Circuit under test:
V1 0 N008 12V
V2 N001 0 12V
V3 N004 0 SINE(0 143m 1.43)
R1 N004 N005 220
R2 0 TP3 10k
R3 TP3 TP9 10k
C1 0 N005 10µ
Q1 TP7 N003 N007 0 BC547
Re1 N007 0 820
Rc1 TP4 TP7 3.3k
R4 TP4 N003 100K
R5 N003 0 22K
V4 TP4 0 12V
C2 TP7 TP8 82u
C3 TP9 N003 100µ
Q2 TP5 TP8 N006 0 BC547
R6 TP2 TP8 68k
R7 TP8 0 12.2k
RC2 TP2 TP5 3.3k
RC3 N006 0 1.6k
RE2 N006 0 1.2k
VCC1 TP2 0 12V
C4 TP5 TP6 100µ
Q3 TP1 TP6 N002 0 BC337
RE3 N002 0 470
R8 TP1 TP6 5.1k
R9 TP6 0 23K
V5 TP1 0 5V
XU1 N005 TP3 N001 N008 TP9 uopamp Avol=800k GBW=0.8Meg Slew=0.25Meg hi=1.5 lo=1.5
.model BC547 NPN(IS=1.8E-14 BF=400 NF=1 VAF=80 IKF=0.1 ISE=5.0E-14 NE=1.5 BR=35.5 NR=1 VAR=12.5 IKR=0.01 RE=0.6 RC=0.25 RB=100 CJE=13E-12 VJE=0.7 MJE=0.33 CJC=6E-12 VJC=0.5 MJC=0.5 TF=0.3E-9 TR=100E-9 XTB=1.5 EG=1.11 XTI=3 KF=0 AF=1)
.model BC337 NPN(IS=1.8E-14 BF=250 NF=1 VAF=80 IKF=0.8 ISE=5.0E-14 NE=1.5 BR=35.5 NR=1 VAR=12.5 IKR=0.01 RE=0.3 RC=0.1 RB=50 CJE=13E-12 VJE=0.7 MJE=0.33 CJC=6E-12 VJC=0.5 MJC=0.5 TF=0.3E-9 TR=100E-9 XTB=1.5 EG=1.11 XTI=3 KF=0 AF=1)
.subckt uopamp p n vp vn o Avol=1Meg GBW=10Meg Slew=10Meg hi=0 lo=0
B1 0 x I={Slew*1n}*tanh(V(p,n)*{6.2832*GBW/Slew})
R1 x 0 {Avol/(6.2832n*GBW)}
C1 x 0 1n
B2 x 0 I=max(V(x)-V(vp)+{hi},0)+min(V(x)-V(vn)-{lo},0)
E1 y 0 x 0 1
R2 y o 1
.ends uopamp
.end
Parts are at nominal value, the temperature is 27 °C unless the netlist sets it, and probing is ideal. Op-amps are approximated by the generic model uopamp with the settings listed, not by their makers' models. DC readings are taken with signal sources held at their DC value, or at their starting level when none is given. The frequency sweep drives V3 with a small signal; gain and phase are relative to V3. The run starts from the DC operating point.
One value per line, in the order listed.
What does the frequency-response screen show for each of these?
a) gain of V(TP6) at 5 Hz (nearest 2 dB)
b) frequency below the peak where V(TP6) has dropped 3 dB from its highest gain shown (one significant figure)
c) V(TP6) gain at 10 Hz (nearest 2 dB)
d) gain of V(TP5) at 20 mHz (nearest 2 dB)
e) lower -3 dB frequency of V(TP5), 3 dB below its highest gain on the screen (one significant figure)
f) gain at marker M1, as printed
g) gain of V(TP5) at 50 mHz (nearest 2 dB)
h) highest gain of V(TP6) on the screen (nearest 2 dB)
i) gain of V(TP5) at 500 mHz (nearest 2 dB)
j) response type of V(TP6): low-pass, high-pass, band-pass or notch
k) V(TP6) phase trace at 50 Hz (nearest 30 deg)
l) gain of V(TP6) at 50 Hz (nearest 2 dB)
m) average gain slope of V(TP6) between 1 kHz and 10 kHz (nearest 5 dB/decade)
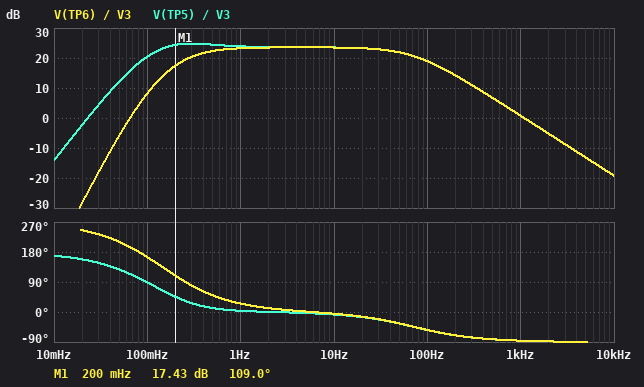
24 dB
300 mHz
24 dB
-2 dB
100 mHz
17.43 dB
12 dB
24 dB
24 dB
band-pass
-30 deg
22 dB
-20 dB/decade
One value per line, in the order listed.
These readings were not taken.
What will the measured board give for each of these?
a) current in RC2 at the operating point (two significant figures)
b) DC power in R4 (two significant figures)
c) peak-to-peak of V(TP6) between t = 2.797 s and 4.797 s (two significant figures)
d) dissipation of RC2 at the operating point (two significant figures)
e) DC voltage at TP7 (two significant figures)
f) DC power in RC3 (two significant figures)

1.6 mA
990 µW
3.9 V
8.7 mW
6.3 V
780 µW
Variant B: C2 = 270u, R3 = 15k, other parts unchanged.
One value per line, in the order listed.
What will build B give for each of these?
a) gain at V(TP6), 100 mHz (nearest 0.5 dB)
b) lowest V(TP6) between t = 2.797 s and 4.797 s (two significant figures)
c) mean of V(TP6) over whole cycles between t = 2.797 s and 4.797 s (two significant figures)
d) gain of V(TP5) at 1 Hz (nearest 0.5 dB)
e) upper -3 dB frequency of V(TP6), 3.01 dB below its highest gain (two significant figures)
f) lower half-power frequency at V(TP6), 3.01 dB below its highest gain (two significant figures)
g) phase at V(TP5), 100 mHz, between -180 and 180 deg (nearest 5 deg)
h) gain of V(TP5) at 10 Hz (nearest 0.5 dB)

14.5 dB
1.2 V
3.7 V
26.0 dB
73 Hz
260 mHz
55 deg
25.5 dB
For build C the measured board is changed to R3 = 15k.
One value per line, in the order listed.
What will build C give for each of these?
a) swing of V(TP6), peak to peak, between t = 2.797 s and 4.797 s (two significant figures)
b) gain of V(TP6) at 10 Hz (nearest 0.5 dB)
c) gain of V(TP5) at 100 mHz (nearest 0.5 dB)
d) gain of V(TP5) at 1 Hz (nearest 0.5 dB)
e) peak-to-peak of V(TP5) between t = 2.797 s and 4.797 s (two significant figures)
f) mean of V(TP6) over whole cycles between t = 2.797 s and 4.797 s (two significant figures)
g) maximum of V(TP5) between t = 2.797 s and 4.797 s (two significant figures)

4.5 V
25.5 dB
22.5 dB
26.0 dB
5.2 V
3.7 V
9.1 V
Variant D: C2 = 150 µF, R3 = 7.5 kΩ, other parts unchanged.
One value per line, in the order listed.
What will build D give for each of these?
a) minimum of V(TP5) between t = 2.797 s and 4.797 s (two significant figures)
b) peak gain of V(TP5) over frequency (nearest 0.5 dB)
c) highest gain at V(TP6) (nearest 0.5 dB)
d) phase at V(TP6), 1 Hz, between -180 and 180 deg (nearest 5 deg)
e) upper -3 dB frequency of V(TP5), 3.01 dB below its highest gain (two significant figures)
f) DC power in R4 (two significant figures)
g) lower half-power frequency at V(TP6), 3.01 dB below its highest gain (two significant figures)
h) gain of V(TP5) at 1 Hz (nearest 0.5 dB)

4.7 V
24.5 dB
22.5 dB
20 deg
36 Hz
990 µW
270 mHz
23.0 dB
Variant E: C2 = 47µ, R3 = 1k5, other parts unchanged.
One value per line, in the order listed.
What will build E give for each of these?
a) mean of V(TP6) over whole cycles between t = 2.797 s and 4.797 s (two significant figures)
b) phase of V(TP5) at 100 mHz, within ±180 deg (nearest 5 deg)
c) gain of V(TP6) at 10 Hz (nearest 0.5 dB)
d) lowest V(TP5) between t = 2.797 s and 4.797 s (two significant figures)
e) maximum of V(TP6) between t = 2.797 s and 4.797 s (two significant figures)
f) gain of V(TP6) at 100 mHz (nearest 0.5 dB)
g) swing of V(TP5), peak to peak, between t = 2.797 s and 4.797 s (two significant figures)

4.0 V
100 deg
18.5 dB
5.4 V
5.2 V
-0.5 dB
2.5 V
